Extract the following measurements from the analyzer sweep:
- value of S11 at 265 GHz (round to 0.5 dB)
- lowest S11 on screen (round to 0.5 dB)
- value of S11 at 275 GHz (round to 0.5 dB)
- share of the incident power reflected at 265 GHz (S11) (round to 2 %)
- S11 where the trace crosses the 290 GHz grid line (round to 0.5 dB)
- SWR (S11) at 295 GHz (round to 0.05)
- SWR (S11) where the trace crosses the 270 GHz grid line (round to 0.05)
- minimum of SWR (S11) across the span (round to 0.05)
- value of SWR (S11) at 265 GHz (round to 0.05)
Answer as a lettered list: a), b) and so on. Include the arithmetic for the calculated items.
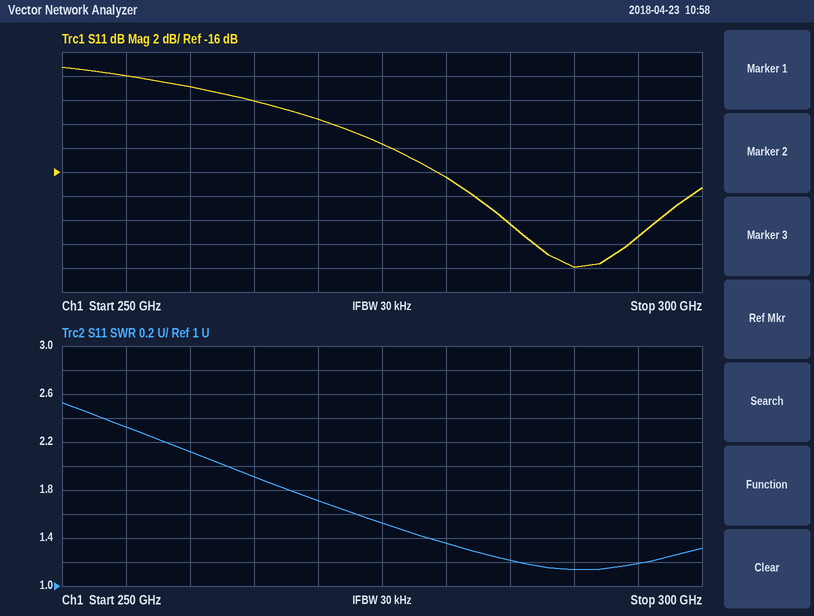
a) -10.0 dB
b) -24.0 dB
c) -13.5 dB
d) 10^(-10/10) ≈ 10 %
e) -24.0 dB
f) 1.20
g) 1.70
h) 1.15
i) 1.90
